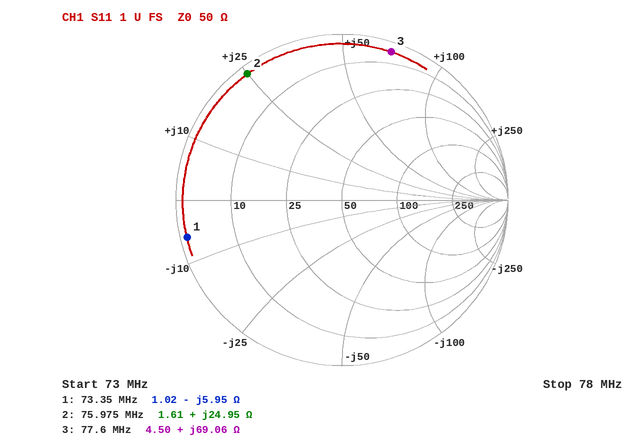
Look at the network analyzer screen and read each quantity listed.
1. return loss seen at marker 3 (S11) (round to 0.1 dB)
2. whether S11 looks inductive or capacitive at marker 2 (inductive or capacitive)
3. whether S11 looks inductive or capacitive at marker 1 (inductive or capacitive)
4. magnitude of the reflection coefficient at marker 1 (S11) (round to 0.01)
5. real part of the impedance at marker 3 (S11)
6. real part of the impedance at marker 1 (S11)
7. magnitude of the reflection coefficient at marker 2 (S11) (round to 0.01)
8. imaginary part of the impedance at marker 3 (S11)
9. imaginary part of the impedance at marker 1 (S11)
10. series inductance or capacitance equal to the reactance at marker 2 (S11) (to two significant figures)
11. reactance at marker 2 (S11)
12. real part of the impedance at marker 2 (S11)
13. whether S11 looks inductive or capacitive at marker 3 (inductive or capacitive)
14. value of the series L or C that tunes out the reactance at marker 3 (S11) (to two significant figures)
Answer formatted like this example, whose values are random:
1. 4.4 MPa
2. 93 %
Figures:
1. 0.5 dB
2. inductive
3. capacitive
4. 0.96
5. 4.50 Ω
6. 1.02 Ω
7. 0.95
8. +69.06 Ω
9. -5.95 Ω
10. 52 nH
11. +24.95 Ω
12. 1.61 Ω
13. inductive
14. 30 pF
